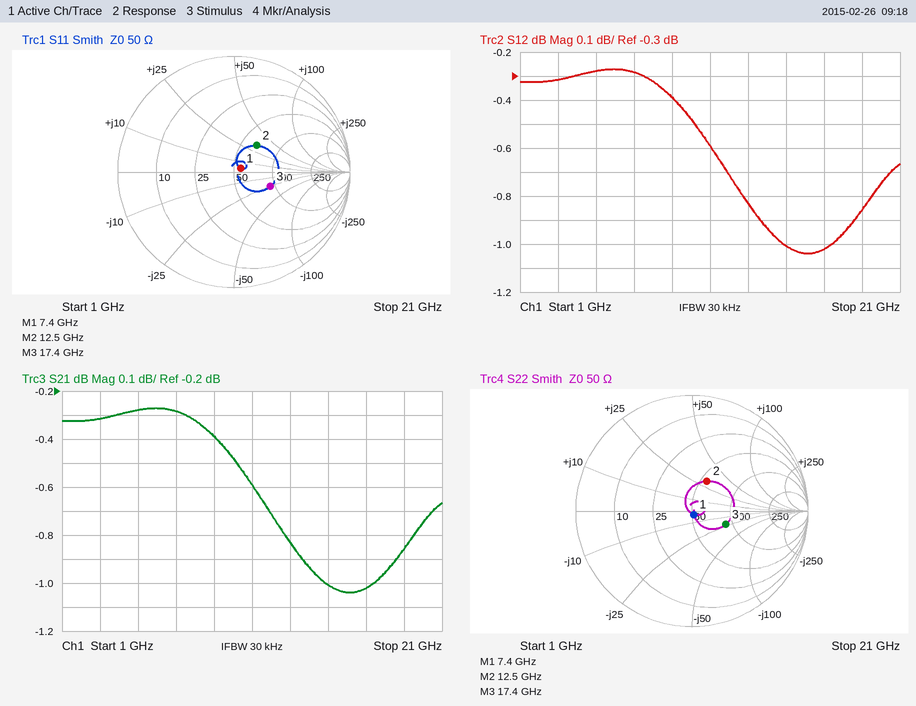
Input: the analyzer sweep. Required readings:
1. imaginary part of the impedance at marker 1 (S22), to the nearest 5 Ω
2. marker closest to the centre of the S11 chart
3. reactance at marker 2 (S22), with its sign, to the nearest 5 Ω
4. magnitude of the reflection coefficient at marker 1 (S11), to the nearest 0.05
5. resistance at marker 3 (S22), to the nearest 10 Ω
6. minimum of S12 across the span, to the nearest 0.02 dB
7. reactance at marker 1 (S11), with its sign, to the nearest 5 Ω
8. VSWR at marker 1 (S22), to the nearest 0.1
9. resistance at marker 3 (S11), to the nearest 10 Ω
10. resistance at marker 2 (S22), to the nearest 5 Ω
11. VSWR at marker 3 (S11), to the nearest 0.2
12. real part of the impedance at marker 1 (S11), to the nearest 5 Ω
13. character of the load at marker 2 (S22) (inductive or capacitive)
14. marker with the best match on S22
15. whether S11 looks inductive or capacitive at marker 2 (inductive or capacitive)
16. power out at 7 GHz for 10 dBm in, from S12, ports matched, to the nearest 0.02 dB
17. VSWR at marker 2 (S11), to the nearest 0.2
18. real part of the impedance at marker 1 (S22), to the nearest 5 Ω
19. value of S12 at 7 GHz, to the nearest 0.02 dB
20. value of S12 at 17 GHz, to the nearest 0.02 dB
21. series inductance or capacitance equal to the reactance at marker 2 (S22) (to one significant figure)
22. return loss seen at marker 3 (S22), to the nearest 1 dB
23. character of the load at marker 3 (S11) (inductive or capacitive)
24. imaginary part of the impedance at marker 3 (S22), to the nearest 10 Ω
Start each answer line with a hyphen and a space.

- -5 Ω
- marker 1
- +30 Ω
- 0.05
- 90 Ω
- -1.04 dB
- +5 Ω
- 1.1
- 90 Ω
- 55 Ω
- 2.0
- 55 Ω
- inductive
- marker 1
- inductive
- 9.72 dBm
- 1.8
- 50 Ω
- -0.28 dB
- -1.02 dB
- 400 pH
- 10 dB
- capacitive
- -20 Ω
